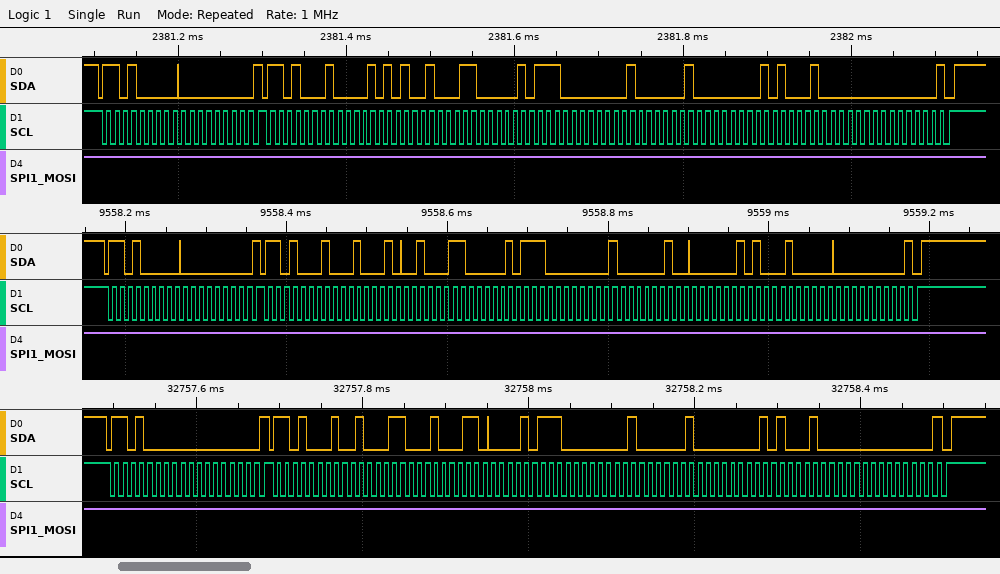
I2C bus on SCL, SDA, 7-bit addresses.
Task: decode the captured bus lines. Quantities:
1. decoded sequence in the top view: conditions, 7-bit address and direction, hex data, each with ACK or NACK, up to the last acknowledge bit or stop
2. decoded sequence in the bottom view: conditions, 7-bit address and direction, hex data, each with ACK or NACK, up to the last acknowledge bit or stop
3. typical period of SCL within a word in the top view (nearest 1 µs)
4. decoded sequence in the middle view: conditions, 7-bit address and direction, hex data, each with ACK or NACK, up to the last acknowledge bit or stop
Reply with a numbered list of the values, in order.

1. start, address 68 write ACK, 00 ACK, repeated start, address 68 read ACK, 15 ACK, 46 ACK, 17 ACK, 01 ACK, 04 ACK, 05 ACK, 20 ACK, 00 NACK, stop
2. start, address 68 write ACK, 00 ACK, repeated start, address 68 read ACK, 46 ACK, 46 ACK, 17 ACK, 01 ACK, 04 ACK, 05 ACK, 20 ACK, 00 NACK, stop
3. 10 µs
4. start, address 68 write ACK, 00 ACK, repeated start, address 68 read ACK, 22 ACK, 46 ACK, 17 ACK, 01 ACK, 04 ACK, 05 ACK, 20 ACK, 00 NACK, stop
